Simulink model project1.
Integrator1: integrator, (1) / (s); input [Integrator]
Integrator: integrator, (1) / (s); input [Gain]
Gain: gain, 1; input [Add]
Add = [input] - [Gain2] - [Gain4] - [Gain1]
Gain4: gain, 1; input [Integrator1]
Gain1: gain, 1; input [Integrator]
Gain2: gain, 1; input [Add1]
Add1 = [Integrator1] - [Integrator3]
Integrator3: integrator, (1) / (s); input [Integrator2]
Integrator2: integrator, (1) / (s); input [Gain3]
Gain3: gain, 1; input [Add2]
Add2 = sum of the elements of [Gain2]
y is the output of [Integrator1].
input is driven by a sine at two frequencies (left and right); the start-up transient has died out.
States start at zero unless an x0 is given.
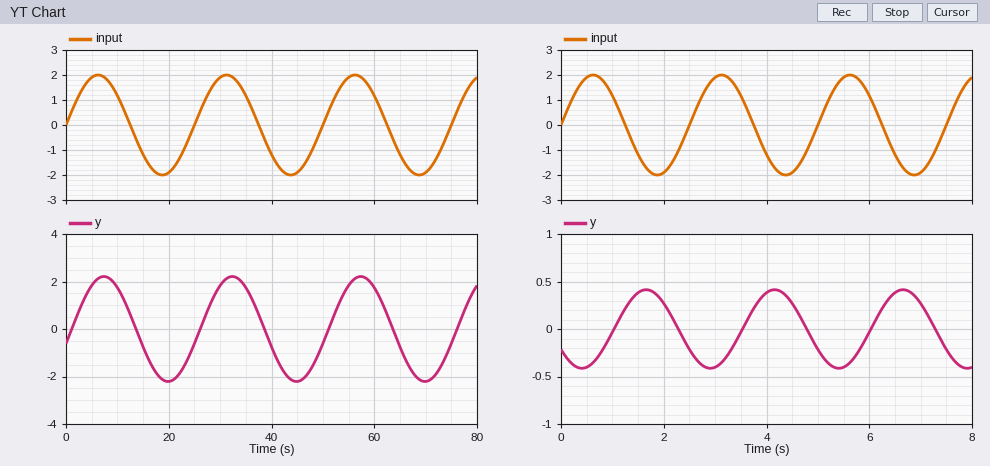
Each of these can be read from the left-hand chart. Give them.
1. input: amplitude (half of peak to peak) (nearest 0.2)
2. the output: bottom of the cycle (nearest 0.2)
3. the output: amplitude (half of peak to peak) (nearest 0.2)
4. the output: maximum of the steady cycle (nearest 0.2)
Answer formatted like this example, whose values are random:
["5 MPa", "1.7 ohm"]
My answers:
["2.0", "-2.2", "2.2", "2.2"]
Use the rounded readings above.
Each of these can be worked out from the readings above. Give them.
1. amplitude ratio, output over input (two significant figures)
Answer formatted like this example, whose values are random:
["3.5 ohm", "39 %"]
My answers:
["1.1"]
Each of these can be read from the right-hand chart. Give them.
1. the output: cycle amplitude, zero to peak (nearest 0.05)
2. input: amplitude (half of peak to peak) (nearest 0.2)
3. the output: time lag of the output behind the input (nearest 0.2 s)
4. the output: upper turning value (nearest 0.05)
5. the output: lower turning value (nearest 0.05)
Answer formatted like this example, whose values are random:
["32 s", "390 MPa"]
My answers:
["0.40", "2.0", "1.0 s", "0.40", "-0.40"]
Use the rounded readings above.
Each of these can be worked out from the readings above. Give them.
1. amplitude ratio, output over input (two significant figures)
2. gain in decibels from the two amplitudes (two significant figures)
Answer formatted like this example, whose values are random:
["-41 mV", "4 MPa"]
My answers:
["0.20", "-14 dB"]
